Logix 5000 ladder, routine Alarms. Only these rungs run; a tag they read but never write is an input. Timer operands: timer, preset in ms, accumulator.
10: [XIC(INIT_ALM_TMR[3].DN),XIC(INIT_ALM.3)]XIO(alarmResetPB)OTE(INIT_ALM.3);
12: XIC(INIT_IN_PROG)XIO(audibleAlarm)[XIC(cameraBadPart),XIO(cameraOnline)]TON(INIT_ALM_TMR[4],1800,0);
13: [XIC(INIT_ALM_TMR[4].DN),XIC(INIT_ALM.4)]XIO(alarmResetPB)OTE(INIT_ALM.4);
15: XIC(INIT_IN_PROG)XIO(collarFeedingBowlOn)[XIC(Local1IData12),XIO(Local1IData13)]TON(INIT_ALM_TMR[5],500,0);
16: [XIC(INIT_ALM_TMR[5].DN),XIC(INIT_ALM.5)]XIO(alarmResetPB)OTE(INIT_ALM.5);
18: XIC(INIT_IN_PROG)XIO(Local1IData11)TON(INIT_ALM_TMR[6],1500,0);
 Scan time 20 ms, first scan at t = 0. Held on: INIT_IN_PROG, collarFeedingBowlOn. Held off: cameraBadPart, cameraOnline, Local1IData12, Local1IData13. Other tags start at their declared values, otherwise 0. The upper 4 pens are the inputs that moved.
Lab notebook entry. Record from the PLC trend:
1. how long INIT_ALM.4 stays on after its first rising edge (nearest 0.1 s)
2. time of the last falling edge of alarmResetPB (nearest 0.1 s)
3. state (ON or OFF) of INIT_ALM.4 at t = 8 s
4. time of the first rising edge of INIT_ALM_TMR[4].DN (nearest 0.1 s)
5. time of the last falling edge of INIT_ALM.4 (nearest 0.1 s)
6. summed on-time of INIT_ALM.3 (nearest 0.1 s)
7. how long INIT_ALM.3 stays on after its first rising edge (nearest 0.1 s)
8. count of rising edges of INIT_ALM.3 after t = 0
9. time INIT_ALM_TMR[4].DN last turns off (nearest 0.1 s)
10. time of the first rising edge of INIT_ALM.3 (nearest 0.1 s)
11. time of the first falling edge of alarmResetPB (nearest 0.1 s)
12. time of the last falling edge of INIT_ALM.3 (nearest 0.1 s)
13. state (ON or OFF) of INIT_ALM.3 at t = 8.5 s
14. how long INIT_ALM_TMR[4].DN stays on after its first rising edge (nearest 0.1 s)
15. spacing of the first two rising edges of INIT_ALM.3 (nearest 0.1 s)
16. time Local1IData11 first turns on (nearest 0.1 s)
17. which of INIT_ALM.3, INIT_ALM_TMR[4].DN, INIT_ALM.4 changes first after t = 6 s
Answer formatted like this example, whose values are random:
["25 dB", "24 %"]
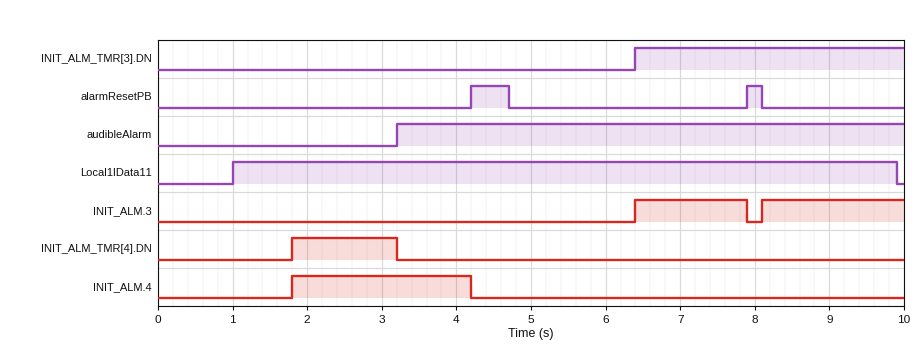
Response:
["2.4 s", "8.1 s", "OFF", "1.8 s", "4.2 s", "3.4 s", "1.5 s", "2", "3.2 s", "6.4 s", "4.7 s", "7.9 s", "ON", "1.4 s", "1.7 s", "1.0 s", "INIT_ALM.3"]
